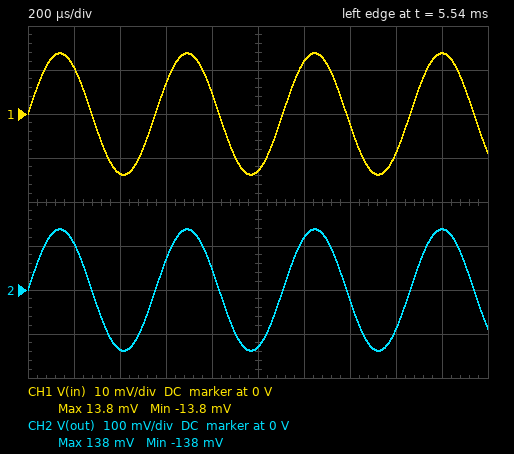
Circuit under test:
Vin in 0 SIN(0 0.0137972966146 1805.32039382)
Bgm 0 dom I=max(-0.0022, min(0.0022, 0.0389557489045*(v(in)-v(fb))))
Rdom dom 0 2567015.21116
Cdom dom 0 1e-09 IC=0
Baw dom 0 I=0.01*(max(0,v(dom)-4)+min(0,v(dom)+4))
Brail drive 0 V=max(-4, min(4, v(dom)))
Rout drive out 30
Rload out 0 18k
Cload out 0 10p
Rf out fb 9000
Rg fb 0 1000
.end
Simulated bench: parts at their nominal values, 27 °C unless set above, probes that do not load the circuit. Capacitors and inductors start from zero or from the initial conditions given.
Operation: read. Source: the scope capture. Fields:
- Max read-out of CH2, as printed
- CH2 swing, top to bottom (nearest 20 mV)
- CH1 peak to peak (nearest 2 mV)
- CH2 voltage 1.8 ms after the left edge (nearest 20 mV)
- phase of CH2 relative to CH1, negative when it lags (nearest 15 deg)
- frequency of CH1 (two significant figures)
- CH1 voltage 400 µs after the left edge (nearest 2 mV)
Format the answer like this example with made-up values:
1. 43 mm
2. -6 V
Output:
1. 138 mV
2. 280 mV
3. 28 mV
4. 140 mV
5. 0 deg
6. 1.8 kHz
7. -14 mV
